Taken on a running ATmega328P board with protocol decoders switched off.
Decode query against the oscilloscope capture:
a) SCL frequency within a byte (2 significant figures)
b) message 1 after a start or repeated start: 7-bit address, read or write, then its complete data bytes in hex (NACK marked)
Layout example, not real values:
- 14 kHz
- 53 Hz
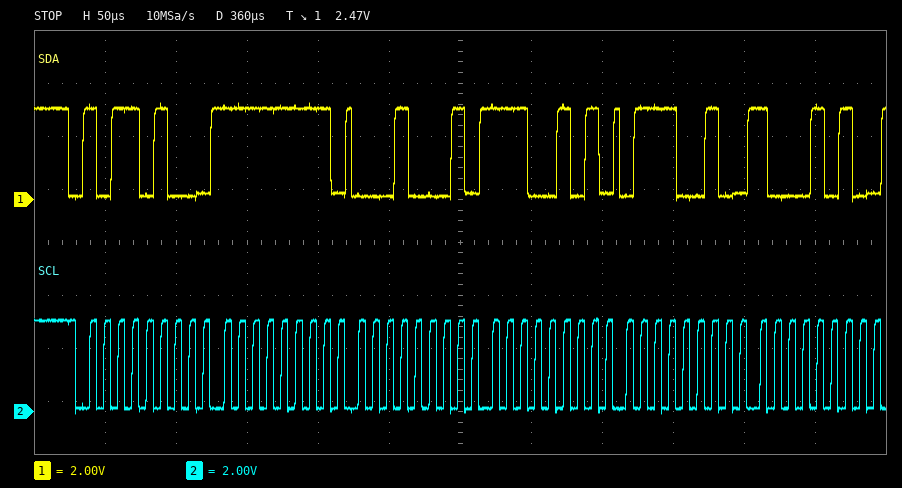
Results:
- 100 kHz
- 0x5A write: FF 11 E5 72 8A
